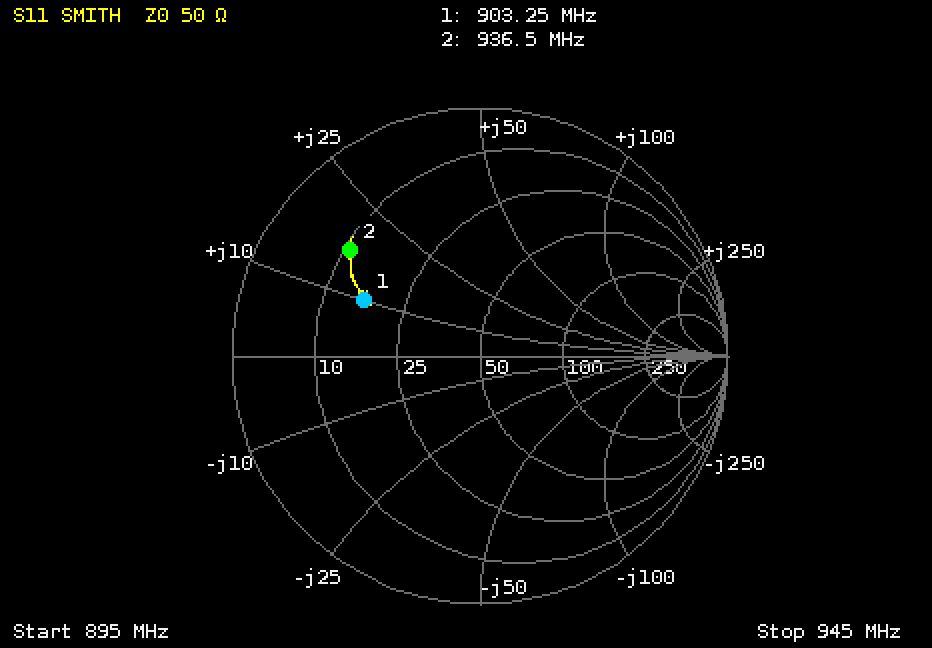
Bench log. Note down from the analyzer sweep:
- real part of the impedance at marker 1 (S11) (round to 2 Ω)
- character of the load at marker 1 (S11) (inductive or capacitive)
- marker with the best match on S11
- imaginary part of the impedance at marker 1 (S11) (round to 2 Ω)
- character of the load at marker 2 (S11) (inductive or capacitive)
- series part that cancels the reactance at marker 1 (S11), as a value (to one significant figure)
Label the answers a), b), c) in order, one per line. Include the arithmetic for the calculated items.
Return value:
a) 16 Ω
b) inductive
c) marker 1
d) +10 Ω
e) inductive
f) C = 1/(2π × 903.25 MHz × 10 Ω) ≈ 17.6 pF, so 20 pF to one significant figure
